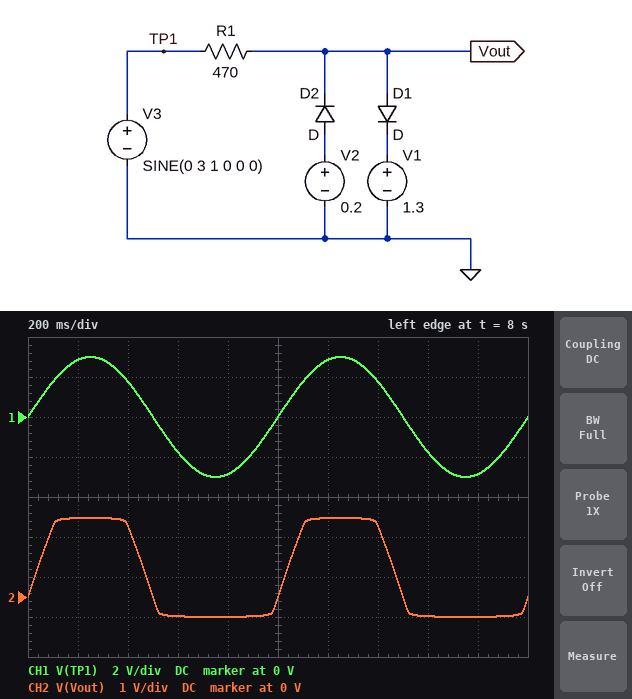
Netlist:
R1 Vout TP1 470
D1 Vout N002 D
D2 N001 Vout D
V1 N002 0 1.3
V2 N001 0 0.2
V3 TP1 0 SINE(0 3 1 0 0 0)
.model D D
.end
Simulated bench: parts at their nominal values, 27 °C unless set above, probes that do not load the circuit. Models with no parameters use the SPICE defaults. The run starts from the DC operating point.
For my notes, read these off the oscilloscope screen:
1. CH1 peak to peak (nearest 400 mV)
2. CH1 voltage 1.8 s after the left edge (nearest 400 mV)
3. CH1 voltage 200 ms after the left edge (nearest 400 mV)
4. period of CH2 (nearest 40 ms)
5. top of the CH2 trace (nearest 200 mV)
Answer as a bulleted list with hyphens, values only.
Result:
- 6.0 V
- -2.8 V
- 2.8 V
- 1.00 s
- 2.0 V
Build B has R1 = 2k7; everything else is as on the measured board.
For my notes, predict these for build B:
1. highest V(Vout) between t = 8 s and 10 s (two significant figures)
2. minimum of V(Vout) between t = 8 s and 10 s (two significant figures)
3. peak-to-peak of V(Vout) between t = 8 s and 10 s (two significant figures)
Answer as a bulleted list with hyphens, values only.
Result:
- 1.9 V
- -450 mV
- 2.4 V
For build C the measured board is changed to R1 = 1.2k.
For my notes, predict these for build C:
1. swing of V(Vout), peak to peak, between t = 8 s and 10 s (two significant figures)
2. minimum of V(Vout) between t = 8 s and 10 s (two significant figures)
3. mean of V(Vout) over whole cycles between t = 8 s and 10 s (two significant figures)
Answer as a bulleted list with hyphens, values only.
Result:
- 2.4 V
- -470 mV
- 540 mV
